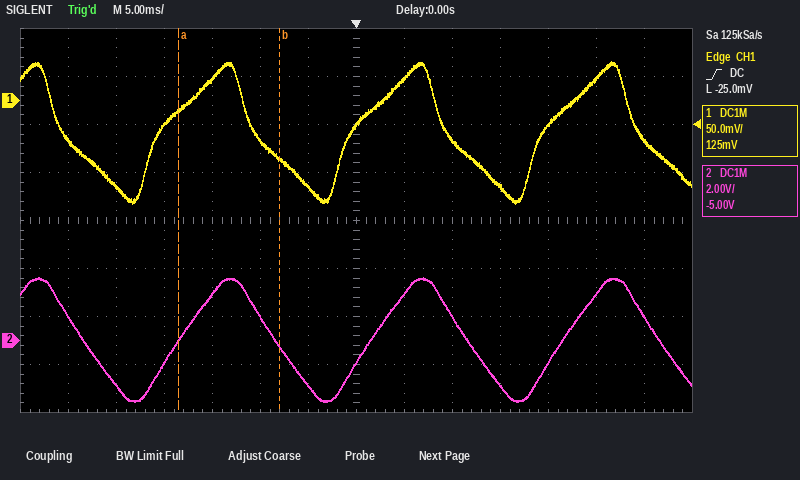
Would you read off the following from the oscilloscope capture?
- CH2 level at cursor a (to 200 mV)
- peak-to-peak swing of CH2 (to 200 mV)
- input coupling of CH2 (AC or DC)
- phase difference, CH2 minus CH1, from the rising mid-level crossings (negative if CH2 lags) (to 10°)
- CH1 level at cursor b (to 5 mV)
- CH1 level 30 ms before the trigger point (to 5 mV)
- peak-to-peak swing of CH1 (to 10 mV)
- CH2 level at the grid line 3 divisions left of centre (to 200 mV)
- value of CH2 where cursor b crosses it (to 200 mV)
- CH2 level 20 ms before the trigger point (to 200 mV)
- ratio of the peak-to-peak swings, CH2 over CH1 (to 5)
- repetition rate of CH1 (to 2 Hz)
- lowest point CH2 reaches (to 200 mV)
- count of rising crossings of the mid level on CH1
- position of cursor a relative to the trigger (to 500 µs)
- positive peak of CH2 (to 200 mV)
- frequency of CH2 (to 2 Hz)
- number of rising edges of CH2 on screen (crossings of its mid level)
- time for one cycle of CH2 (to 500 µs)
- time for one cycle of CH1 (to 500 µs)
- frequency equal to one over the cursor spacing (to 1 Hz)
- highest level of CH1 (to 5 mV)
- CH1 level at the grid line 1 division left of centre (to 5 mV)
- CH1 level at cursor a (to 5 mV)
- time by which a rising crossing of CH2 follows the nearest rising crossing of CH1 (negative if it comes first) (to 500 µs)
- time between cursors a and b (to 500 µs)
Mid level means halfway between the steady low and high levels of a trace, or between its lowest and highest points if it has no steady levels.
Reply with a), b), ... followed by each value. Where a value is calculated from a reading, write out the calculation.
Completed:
a) 0.0 V
b) 2.6 V − (-2.6 V) = 5.2 V
c) DC
d) −360° × (+2.0 ms) / 20.0 ms ≈ -36.0°, so -40° to the nearest 10°
e) -60 mV
f) -40 mV
g) 150 mV
h) 2.0 V
i) -200 mV
j) -1.0 V
k) 5.2 V / 150 mV ≈ 35
l) 1 / 20.0 ms ≈ 50 Hz
m) -2.6 V
n) 3
o) -18.5 ms
p) 2.6 V
q) 1 / 20.0 ms ≈ 50 Hz
r) 3
s) 20.0 ms
t) 20.0 ms
u) 1 / 10.5 ms ≈ 95 Hz
v) 40 mV
w) -90 mV
x) -10 mV
y) +2.0 ms
z) 10.5 ms
